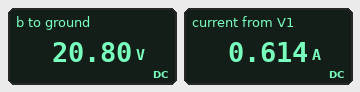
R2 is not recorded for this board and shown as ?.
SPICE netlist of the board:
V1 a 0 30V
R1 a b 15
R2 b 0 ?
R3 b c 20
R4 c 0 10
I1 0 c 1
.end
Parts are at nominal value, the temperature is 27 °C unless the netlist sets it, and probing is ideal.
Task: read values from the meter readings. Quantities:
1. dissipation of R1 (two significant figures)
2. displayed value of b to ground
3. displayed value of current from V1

5.6 W
20.80 V
0.614 A
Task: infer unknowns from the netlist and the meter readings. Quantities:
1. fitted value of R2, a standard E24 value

82 Ω
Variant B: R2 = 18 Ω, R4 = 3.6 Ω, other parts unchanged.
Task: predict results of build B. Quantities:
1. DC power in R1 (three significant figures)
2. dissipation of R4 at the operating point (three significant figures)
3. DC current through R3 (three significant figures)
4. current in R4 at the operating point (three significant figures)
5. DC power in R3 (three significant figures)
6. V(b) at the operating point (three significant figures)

19.1 W
7.07 W
402 mA
1.40 A
3.23 W
13.1 V
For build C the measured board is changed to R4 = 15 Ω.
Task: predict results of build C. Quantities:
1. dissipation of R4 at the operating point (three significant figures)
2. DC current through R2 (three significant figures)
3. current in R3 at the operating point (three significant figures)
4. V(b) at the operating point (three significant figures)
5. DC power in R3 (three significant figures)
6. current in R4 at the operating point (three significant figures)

22.2 W
276 mA
217 mA
22.6 V
944 mW
1.22 A
